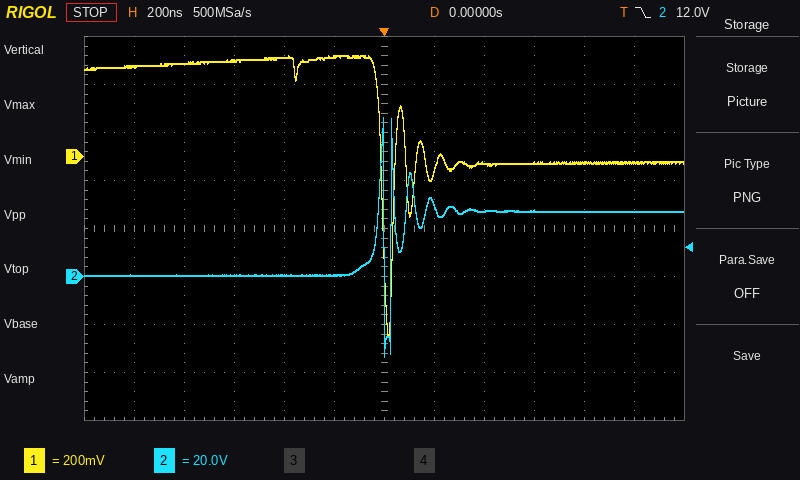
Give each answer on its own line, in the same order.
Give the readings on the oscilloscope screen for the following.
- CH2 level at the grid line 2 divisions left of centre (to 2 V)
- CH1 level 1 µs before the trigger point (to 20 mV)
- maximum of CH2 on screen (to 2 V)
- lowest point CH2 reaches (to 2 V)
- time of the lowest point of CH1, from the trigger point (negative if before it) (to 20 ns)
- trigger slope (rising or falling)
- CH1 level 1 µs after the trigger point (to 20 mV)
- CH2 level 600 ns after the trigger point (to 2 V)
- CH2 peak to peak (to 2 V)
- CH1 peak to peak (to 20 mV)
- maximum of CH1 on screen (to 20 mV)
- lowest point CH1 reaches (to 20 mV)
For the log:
0 V
380 mV
66 V
-34 V
+20 ns
falling
-20 mV
28 V
100 V
1.16 V
420 mV
-740 mV
